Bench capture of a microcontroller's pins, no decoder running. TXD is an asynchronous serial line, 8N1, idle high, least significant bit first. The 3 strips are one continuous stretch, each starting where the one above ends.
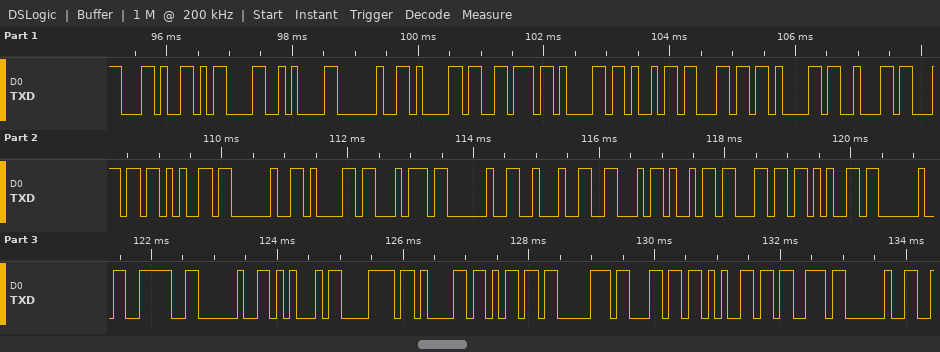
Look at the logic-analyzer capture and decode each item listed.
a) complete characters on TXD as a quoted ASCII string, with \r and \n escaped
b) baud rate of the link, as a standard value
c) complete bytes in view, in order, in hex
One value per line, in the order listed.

",\r\n available at \"File > Examples "
9600 baud
2C 0D 0A 20 61 76 61 69 6C 61 62 6C 65 20 61 74 20 22 46 69 6C 65 20 3E 20 45 78 61 6D 70 6C 65 73 20
